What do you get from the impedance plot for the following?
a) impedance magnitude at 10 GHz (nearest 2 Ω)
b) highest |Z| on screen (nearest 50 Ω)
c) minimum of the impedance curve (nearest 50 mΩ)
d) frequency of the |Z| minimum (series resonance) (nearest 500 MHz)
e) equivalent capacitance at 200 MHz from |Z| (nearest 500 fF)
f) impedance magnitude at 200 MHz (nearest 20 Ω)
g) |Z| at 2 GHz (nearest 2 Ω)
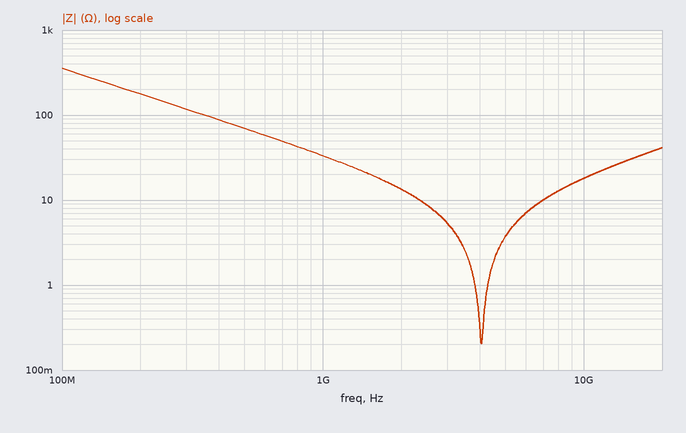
18 Ω
350 Ω
200 mΩ
4.0 GHz
4.5 pF
180 Ω
14 Ω
